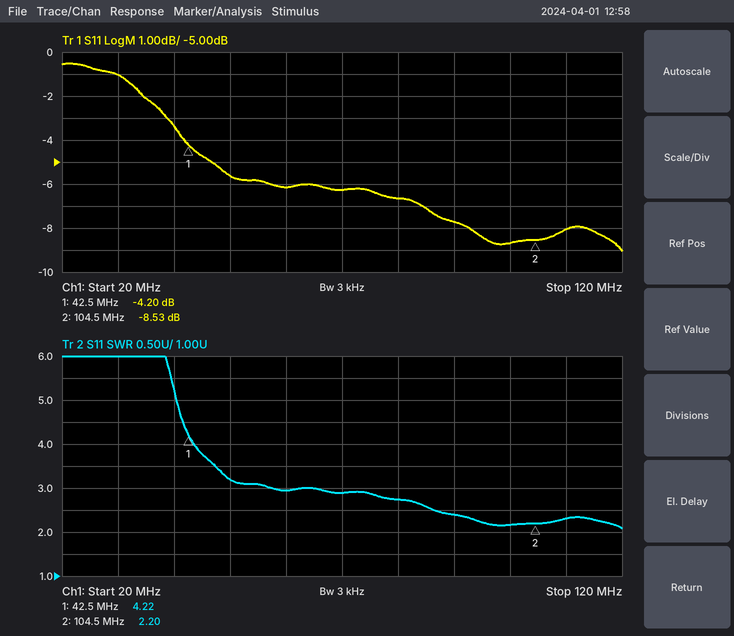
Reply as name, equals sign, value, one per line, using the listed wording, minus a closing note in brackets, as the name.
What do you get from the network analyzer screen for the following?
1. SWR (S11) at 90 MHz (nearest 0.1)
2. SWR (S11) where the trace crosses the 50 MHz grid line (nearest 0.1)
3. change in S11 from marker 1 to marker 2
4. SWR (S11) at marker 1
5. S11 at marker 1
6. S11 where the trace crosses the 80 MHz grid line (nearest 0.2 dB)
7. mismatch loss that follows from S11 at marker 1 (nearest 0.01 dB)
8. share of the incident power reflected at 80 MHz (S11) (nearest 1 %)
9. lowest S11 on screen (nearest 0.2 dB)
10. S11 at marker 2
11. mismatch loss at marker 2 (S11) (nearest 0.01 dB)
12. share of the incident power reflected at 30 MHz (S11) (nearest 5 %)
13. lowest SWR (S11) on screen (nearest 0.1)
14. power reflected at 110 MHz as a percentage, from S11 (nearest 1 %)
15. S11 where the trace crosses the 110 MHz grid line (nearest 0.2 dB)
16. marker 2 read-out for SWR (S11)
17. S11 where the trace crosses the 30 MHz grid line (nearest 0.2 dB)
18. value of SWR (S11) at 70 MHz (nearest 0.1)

SWR (S11) at 90 MHz = 2.4
SWR (S11) where the trace crosses the 50 MHz grid line = 3.2
change in S11 from marker 1 to marker 2 = -4.33 dB
SWR (S11) at marker 1 = 4.22
S11 at marker 1 = -4.20 dB
S11 where the trace crosses the 80 MHz grid line = -6.6 dB
mismatch loss that follows from S11 at marker 1 = 2.08 dB
share of the incident power reflected at 80 MHz (S11) = 22 %
lowest S11 on screen = -9.0 dB
S11 at marker 2 = -8.53 dB
mismatch loss at marker 2 (S11) = 0.66 dB
share of the incident power reflected at 30 MHz (S11) = 80 %
lowest SWR (S11) on screen = 2.1
power reflected at 110 MHz as a percentage, from S11 = 16 %
S11 where the trace crosses the 110 MHz grid line = -8.0 dB
marker 2 read-out for SWR = 2.20
S11 where the trace crosses the 30 MHz grid line = -1.0 dB
value of SWR (S11) at 70 MHz = 2.9
